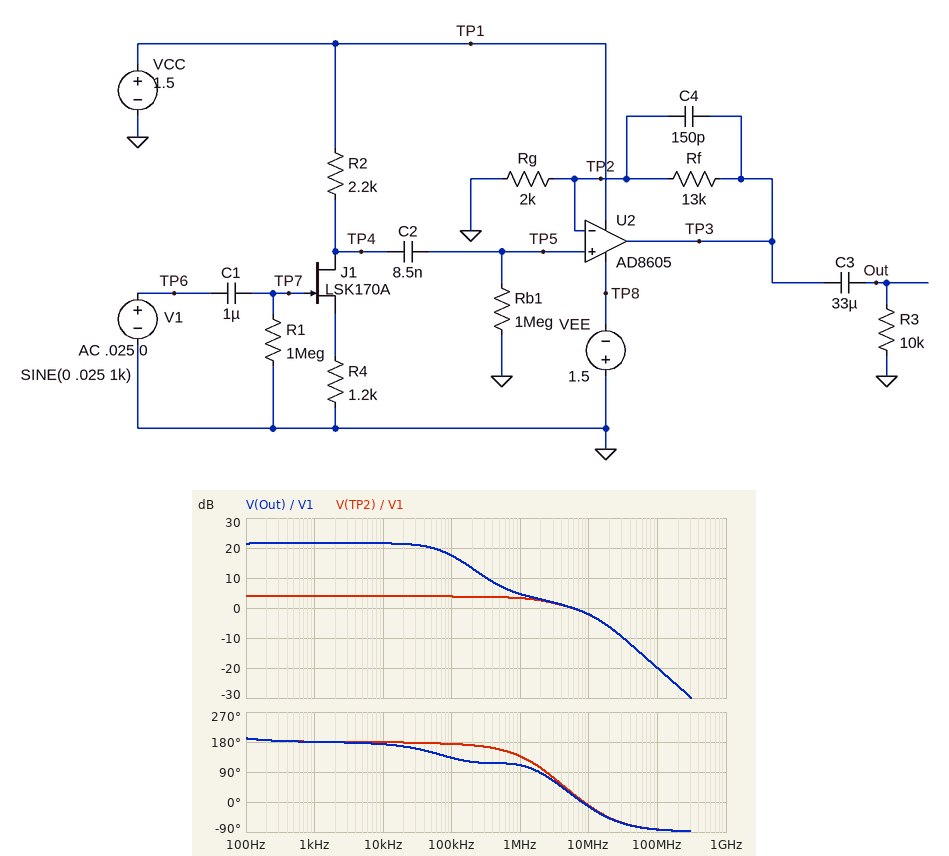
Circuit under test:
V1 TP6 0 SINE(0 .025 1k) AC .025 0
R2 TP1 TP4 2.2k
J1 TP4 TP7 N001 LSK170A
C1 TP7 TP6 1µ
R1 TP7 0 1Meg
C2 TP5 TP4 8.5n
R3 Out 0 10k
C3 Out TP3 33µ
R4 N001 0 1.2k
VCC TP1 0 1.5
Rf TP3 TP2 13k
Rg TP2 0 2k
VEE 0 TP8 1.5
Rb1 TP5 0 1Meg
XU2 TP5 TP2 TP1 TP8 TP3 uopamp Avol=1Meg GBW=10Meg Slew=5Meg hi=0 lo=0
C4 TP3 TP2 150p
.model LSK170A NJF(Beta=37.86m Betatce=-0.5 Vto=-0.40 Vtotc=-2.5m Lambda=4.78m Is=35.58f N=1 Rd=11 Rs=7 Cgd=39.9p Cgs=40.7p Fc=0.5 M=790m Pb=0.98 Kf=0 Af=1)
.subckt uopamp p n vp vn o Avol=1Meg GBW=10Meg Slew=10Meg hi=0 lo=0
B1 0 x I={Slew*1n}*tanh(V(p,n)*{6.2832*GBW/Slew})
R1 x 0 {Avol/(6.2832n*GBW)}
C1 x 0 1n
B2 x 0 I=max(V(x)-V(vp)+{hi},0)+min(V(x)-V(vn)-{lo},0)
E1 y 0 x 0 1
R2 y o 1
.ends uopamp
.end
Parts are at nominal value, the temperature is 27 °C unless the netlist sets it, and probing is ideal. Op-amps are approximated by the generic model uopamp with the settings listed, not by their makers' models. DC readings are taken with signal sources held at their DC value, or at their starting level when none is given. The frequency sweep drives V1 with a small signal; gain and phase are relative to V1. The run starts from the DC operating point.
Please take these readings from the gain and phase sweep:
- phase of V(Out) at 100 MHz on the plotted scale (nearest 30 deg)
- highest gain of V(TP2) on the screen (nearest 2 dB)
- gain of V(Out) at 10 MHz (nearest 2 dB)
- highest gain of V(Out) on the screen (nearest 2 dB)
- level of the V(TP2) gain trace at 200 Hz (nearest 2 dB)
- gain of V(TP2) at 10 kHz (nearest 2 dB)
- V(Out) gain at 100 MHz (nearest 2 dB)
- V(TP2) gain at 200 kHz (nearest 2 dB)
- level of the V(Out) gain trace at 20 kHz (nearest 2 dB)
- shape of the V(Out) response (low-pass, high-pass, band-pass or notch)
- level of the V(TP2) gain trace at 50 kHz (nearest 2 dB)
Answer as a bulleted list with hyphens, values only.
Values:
- -90 deg
- 4 dB
- -2 dB
- 22 dB
- 4 dB
- 4 dB
- -20 dB
- 4 dB
- 22 dB
- low-pass
- 4 dB
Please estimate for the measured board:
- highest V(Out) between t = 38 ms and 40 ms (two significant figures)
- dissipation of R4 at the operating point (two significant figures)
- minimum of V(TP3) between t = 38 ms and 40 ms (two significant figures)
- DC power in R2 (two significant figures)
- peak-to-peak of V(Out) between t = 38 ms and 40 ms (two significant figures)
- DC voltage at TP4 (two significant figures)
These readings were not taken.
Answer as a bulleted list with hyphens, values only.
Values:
- 300 mV
- 83 µW
- -300 mV
- 150 µW
- 600 mV
- 920 mV
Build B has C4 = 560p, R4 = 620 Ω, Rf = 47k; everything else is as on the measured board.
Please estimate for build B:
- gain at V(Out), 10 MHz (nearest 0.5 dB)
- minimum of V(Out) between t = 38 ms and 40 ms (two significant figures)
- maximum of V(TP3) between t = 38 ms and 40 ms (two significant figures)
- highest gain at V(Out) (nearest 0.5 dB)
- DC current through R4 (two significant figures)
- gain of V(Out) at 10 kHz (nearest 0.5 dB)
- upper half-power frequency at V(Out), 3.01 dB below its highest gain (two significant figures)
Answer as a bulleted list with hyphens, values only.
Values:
- -1.0 dB
- -1.5 V
- 1.5 V
- 37.0 dB
- 460 µA
- 31.5 dB
- 6.0 kHz
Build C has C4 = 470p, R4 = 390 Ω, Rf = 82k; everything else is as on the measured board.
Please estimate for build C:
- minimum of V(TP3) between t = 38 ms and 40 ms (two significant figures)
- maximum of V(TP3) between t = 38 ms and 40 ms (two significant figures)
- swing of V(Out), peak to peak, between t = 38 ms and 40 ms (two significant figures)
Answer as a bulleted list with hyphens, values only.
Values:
- -270 mV
- 320 mV
- 590 mV
